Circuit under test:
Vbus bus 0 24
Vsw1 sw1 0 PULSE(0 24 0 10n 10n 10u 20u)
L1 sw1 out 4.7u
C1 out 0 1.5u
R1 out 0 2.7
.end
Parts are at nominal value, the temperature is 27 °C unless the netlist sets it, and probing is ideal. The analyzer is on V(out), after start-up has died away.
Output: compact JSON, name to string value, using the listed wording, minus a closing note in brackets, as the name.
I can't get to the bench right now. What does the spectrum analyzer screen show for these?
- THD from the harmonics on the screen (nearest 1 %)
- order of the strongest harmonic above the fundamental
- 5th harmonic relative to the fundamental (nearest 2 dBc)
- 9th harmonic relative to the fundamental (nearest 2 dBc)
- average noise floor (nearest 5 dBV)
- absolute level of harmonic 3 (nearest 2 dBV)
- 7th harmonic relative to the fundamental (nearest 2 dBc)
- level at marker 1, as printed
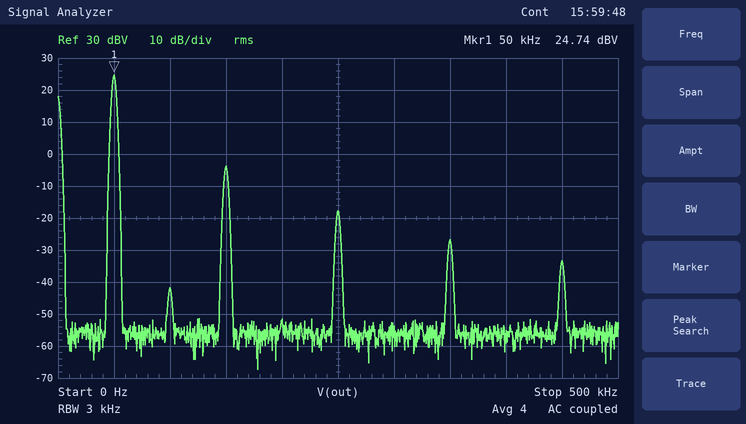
{"THD from the harmonics on the screen": "4 %", "order of the strongest harmonic above the fundamental": "3", "5th harmonic relative to the fundamental": "-42 dBc", "9th harmonic relative to the fundamental": "-58 dBc", "average noise floor": "-55 dBV", "absolute level of harmonic 3": "-4 dBV", "7th harmonic relative to the fundamental": "-52 dBc", "level at marker 1, as printed": "24.74 dBV"}
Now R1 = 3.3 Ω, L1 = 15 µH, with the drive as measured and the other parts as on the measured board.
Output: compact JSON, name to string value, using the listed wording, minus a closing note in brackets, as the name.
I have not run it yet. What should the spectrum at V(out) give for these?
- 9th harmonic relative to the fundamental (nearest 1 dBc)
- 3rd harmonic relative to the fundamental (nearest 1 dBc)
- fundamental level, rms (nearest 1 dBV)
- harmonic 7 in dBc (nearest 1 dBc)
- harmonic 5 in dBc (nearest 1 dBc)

{"9th harmonic relative to the fundamental": "-59 dBc", "3rd harmonic relative to the fundamental": "-30 dBc", "fundamental level, rms": "15 dBV", "harmonic 7 in dBc": "-52 dBc", "harmonic 5 in dBc": "-43 dBc"}
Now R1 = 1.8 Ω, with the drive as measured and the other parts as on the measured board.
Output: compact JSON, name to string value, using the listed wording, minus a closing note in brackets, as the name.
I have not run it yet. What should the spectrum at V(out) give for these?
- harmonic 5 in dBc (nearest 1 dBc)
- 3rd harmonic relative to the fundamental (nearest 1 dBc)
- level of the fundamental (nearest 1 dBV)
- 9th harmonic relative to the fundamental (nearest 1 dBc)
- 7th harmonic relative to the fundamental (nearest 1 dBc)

{"harmonic 5 in dBc": "-40 dBc", "3rd harmonic relative to the fundamental": "-26 dBc", "level of the fundamental": "22 dBV", "9th harmonic relative to the fundamental": "-55 dBc", "7th harmonic relative to the fundamental": "-49 dBc"}
